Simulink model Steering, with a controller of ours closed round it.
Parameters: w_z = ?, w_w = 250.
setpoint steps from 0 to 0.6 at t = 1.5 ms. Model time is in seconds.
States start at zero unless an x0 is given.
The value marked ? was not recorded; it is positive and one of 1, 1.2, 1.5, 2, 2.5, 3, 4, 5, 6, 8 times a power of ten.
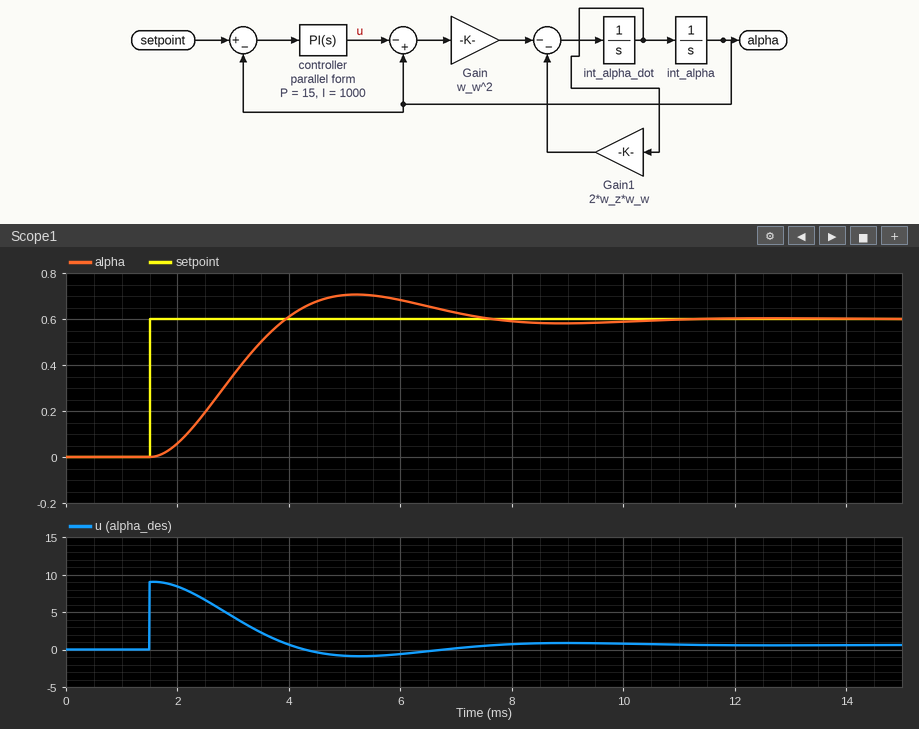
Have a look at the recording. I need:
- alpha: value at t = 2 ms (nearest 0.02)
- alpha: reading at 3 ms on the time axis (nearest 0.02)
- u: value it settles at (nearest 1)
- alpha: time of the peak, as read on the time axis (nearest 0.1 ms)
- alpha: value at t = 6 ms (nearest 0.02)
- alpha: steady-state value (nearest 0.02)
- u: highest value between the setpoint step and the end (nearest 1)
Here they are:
0.06
0.36
1
5.2 ms
0.68
0.60
9
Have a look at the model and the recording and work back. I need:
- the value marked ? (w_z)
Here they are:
2
